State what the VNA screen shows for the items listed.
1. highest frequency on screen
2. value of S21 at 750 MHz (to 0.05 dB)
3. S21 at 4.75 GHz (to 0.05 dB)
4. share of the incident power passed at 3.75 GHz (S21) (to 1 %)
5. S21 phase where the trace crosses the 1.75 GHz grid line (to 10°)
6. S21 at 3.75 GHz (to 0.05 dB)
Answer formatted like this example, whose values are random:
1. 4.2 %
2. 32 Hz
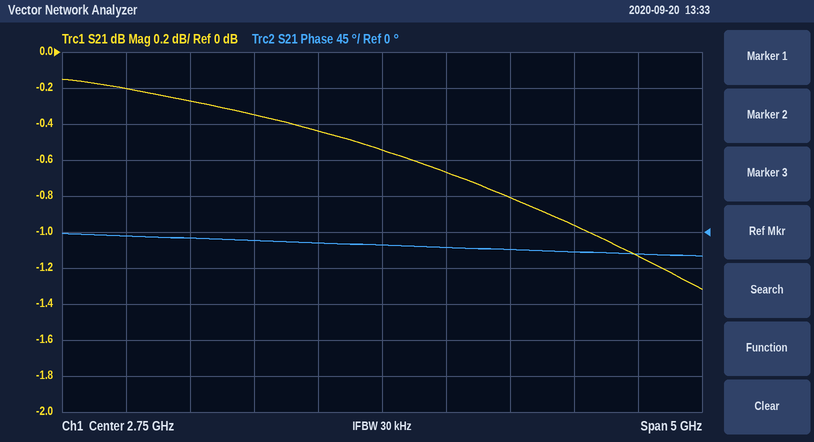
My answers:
1. 5.25 GHz
2. -0.20 dB
3. -1.15 dB
4. 83 %
5. -10°
6. -0.80 dB
